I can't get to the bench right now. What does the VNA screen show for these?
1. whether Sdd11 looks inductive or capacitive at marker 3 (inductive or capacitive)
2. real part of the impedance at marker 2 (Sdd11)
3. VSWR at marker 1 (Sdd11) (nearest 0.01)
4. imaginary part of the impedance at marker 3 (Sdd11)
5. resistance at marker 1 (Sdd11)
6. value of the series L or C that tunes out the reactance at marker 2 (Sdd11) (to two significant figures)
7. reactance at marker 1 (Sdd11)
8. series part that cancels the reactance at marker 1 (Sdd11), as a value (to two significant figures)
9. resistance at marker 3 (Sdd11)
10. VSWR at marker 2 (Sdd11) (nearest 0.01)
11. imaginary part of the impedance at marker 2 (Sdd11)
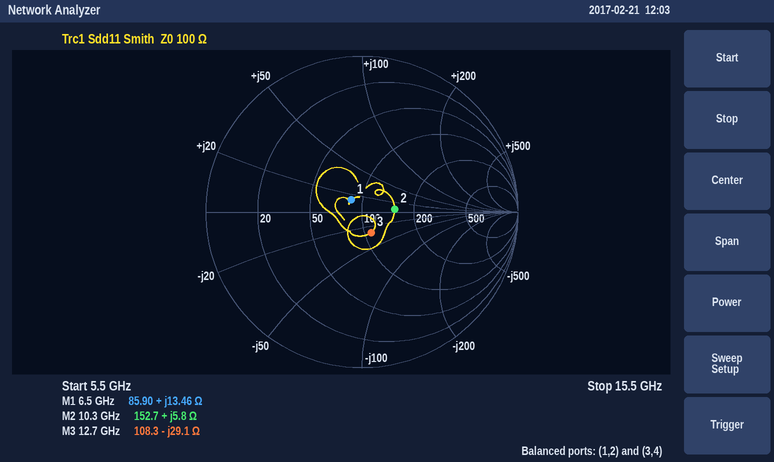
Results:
capacitive
152.7 Ω
1.23
-29.1 Ω
85.90 Ω
2.7 pF
+13.46 Ω
1.8 pF
108.3 Ω
1.53
+5.8 Ω
